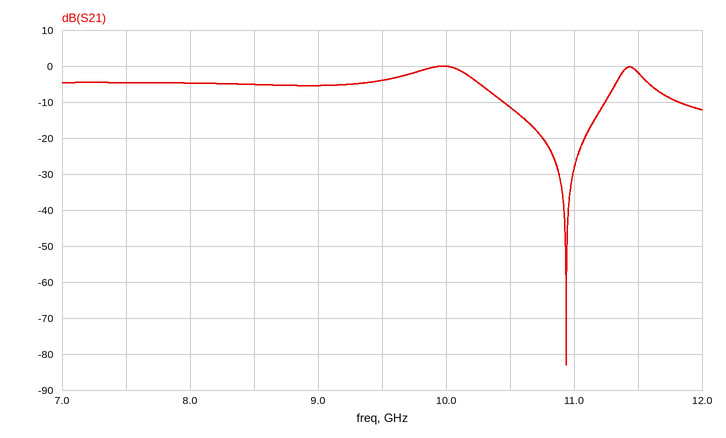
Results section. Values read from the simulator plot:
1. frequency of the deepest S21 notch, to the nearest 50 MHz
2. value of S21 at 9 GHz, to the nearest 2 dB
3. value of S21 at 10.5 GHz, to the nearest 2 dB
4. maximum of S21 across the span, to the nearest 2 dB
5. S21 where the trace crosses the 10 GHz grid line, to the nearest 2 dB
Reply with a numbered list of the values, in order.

1. 10.95 GHz
2. -6 dB
3. -12 dB
4. 0 dB
5. 0 dB
